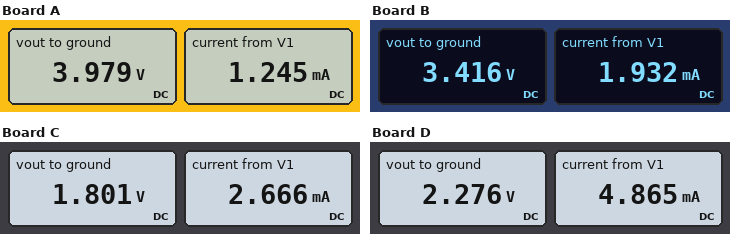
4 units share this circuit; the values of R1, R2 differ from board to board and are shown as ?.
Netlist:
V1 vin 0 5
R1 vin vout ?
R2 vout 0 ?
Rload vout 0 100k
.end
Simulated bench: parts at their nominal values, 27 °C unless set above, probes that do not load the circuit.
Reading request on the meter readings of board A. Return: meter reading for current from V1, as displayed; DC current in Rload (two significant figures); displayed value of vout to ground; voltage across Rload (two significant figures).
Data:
1.245 mA
40 µA
3.979 V
4.0 V
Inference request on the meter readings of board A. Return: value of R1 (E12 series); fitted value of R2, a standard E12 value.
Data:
820 Ω
3.3 kΩ
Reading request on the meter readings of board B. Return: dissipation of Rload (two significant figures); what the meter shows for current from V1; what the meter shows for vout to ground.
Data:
120 µW
1.932 mA
3.416 V
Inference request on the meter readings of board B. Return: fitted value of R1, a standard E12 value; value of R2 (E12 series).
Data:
820 Ω
1.8 kΩ
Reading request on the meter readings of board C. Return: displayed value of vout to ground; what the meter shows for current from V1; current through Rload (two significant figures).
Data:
1.801 V
2.666 mA
18 µA
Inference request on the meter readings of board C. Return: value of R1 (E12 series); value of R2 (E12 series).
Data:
1.2 kΩ
680 Ω
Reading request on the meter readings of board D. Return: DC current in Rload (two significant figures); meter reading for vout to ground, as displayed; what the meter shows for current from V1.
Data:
23 µA
2.276 V
4.865 mA
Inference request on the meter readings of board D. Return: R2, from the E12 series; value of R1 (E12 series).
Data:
470 Ω
560 Ω
